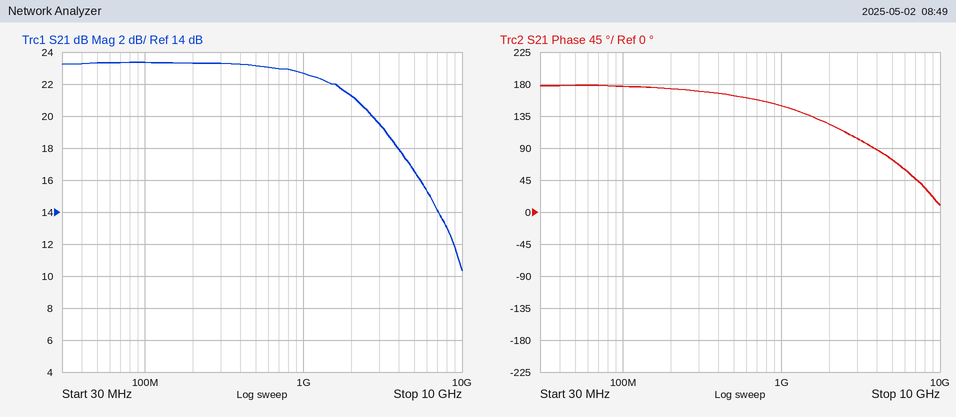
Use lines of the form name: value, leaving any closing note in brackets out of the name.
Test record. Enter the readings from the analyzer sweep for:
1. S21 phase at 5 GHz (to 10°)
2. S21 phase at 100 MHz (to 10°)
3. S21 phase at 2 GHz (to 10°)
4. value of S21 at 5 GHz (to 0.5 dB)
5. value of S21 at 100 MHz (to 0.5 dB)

S21 phase at 5 GHz: 70°
S21 phase at 100 MHz: 180°
S21 phase at 2 GHz: 120°
value of S21 at 5 GHz: 16.5 dB
value of S21 at 100 MHz: 23.5 dB
